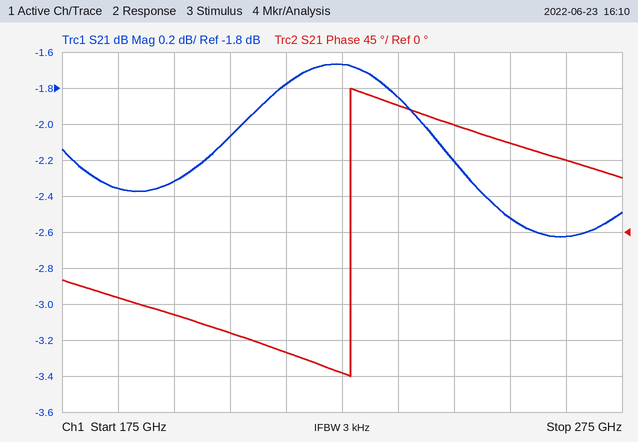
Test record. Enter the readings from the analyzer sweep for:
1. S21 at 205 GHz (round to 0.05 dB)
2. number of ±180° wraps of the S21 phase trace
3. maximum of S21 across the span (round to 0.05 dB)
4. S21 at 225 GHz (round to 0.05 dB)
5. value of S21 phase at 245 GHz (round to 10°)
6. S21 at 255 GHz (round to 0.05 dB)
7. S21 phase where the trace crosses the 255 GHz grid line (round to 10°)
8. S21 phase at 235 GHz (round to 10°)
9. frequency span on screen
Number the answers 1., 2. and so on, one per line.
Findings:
1. -2.05 dB
2. 1
3. -1.65 dB
4. -1.65 dB
5. 130°
6. -2.50 dB
7. 110°
8. 160°
9. 100 GHz
